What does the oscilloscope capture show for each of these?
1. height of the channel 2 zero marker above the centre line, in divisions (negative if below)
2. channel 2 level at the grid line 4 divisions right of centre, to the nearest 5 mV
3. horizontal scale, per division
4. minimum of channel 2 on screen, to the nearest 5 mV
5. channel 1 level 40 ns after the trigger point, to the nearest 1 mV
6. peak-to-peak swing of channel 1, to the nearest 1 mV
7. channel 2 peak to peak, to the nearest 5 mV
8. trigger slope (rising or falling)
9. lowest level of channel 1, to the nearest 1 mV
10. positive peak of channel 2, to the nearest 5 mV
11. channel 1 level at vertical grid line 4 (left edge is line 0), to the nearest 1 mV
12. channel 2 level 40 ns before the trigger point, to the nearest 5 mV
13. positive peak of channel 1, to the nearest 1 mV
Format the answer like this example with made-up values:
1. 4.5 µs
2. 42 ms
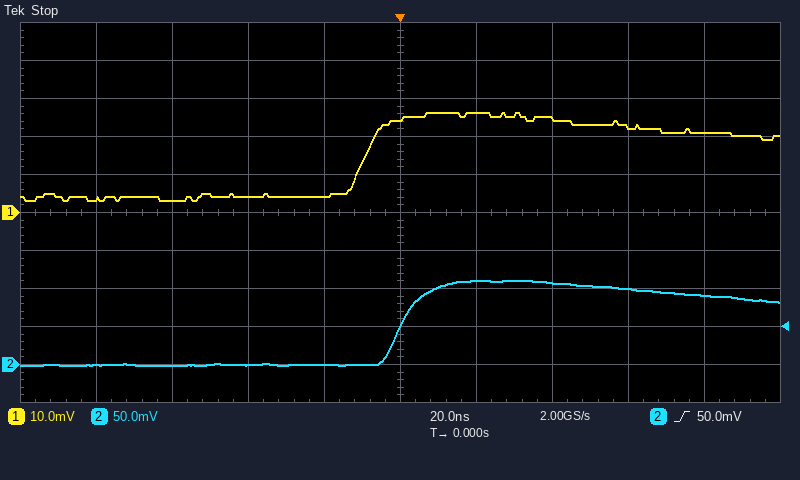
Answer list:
1. -4.0 div
2. 90 mV
3. 20 ns
4. 0 mV
5. 25 mV
6. 23 mV
7. 110 mV
8. rising
9. 3 mV
10. 110 mV
11. 4 mV
12. 0 mV
13. 26 mV
